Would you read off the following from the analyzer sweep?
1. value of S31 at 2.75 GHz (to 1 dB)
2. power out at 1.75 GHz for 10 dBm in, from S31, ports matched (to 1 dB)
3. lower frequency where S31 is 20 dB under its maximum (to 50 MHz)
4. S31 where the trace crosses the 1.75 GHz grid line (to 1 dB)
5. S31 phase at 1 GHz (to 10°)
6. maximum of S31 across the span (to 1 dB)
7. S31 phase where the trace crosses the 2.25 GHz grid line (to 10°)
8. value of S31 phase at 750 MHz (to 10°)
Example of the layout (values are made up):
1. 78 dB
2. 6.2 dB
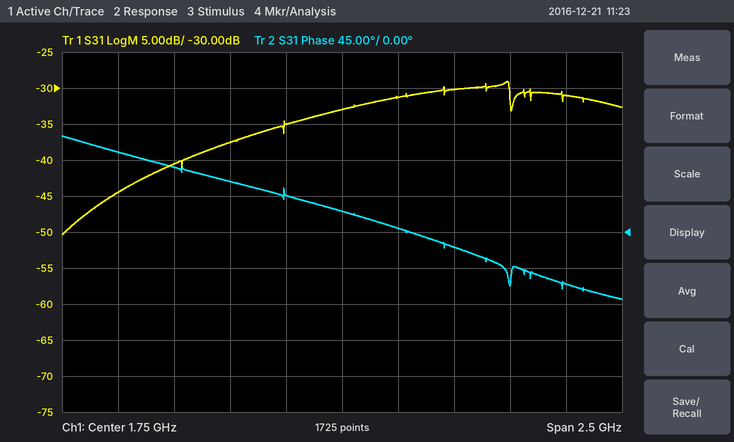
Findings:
1. -31 dB
2. -23 dBm
3. 550 MHz
4. -33 dB
5. 80°
6. -29 dB
7. -20°
8. 100°
